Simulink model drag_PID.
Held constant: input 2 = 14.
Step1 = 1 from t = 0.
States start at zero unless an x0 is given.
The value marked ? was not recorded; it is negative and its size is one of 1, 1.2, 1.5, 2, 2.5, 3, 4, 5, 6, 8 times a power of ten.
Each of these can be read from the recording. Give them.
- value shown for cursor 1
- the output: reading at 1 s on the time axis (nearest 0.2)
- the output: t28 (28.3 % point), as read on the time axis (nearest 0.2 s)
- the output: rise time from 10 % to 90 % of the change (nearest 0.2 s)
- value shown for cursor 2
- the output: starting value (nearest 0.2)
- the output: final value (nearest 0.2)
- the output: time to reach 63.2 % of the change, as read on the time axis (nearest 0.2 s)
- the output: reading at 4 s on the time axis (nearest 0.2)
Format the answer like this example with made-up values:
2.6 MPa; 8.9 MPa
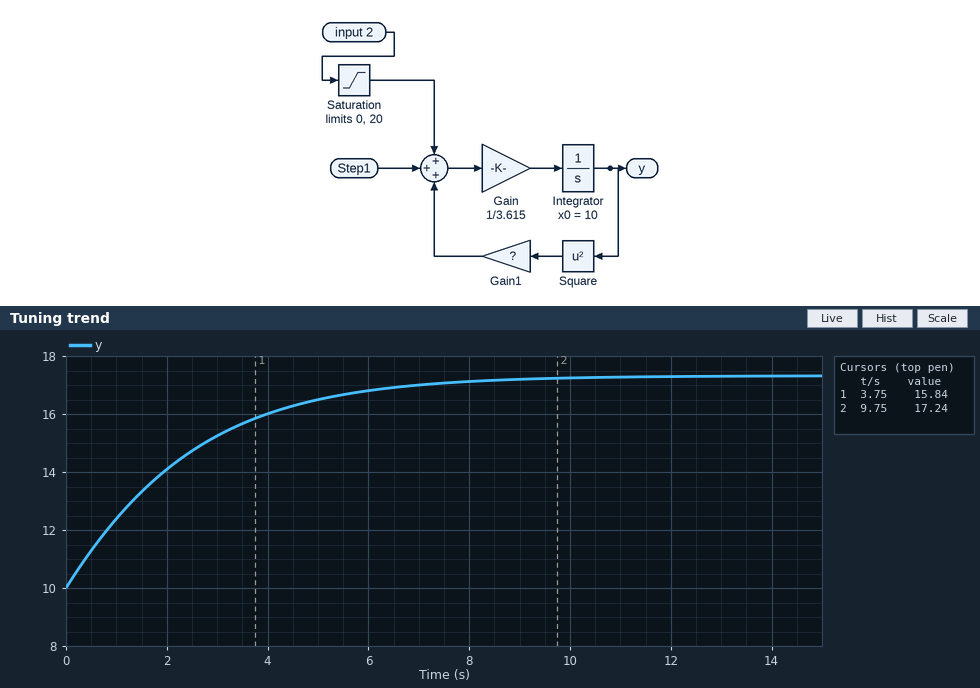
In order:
15.84; 12.4; 0.8 s; 5.0 s; 17.24; 10.0; 17.4; 2.4 s; 16.0
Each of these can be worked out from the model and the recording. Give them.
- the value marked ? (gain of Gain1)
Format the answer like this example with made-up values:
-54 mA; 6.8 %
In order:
-0.05
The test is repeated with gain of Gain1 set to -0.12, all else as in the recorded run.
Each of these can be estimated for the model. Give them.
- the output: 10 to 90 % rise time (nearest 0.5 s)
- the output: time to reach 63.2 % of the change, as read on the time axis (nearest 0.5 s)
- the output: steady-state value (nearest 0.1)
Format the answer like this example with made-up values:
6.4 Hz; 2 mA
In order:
3.0 s; 1.5 s; 11.2
